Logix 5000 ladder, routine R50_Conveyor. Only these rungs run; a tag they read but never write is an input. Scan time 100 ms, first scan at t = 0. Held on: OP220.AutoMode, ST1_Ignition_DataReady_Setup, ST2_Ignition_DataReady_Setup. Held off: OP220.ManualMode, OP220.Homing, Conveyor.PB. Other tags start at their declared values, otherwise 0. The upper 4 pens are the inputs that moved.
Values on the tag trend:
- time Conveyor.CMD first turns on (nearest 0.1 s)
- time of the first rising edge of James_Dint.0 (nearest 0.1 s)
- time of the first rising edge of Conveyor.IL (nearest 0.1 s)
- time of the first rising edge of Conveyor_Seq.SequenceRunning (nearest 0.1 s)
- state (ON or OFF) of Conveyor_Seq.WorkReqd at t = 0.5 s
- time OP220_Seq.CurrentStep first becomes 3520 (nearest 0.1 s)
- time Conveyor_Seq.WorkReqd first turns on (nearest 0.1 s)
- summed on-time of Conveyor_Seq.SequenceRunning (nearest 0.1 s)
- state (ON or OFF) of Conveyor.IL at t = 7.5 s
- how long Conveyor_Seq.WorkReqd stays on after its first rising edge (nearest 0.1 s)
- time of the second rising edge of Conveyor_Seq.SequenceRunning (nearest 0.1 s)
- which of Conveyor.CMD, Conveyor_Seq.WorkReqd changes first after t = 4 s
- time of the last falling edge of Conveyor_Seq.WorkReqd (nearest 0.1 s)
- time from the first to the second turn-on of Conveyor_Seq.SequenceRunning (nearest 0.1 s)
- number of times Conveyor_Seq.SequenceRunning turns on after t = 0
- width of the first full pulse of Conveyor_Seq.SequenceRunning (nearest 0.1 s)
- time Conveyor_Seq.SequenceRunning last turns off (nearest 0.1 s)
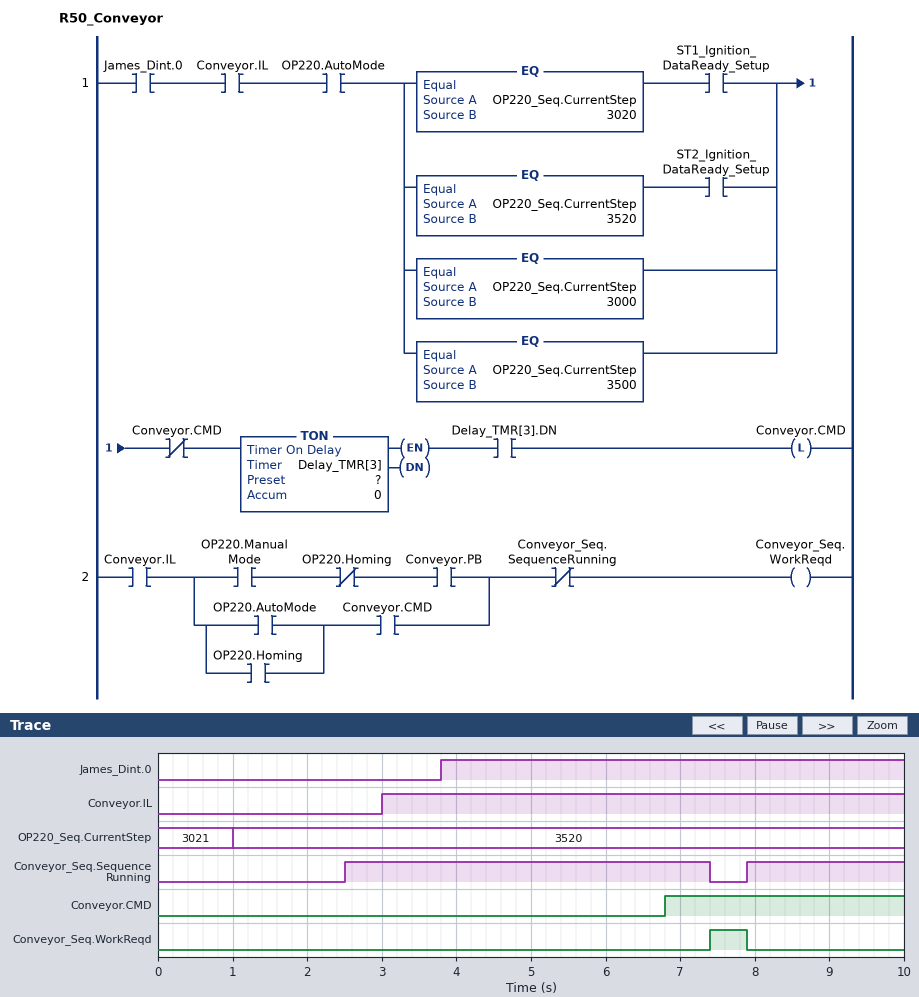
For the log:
6.8 s
3.8 s
3.0 s
2.5 s
OFF
1.0 s
7.4 s
7.0 s
ON
0.5 s
7.9 s
Conveyor.CMD
7.9 s
5.4 s
2
4.9 s
7.4 s
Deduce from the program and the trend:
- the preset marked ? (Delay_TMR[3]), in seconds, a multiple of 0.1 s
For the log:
3.0 s
